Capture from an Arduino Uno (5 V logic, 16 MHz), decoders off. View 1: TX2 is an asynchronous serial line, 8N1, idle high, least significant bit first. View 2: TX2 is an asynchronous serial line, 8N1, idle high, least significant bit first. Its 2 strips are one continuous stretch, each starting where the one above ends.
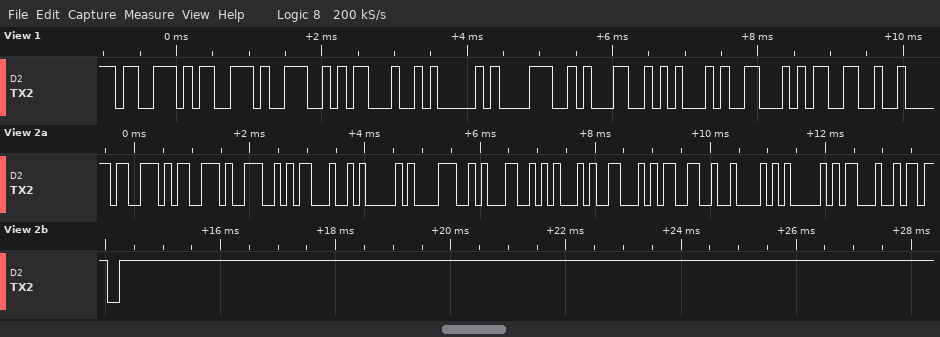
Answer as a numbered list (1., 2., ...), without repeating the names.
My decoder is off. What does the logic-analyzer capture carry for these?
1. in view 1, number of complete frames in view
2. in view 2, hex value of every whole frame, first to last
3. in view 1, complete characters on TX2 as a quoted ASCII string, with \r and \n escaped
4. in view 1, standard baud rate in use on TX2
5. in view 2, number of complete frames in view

1. 10
2. 0x73 0x73 0x4E 0x23 0x41 0x38 0x31 0x45 0x46 0x33 0x42 0x41 0x23 0x3B
3. "ssN#A81EF3"
4. 9600 baud
5. 14
